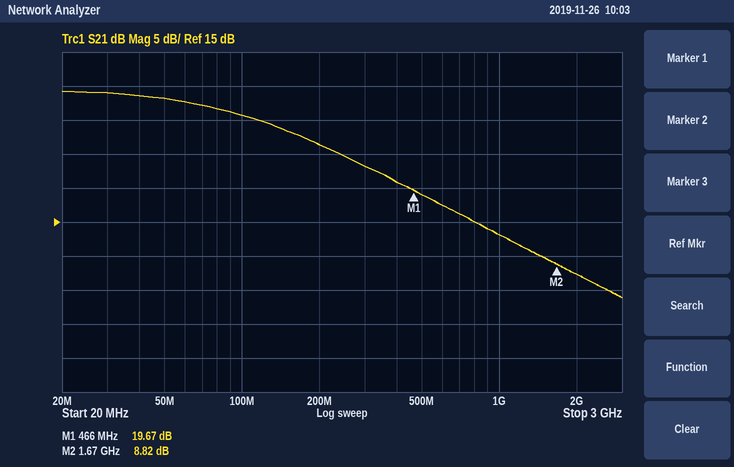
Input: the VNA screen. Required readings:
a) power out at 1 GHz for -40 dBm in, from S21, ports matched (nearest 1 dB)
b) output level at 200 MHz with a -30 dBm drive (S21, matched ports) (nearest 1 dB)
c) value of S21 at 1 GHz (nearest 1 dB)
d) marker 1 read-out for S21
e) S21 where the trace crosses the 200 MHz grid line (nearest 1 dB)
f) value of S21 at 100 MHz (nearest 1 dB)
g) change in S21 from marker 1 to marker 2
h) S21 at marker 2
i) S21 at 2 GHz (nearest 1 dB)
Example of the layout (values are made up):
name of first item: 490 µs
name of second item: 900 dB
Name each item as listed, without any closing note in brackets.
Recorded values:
power out at 1 GHz for -40 dBm in, from S21, ports matched: -27 dBm
output level at 200 MHz with a -30 dBm drive (S21, matched ports): -4 dBm
value of S21 at 1 GHz: 13 dB
marker 1 read-out for S21: 19.67 dB
S21 where the trace crosses the 200 MHz grid line: 26 dB
value of S21 at 100 MHz: 31 dB
change in S21 from marker 1 to marker 2: -10.85 dB
S21 at marker 2: 8.82 dB
S21 at 2 GHz: 7 dB
